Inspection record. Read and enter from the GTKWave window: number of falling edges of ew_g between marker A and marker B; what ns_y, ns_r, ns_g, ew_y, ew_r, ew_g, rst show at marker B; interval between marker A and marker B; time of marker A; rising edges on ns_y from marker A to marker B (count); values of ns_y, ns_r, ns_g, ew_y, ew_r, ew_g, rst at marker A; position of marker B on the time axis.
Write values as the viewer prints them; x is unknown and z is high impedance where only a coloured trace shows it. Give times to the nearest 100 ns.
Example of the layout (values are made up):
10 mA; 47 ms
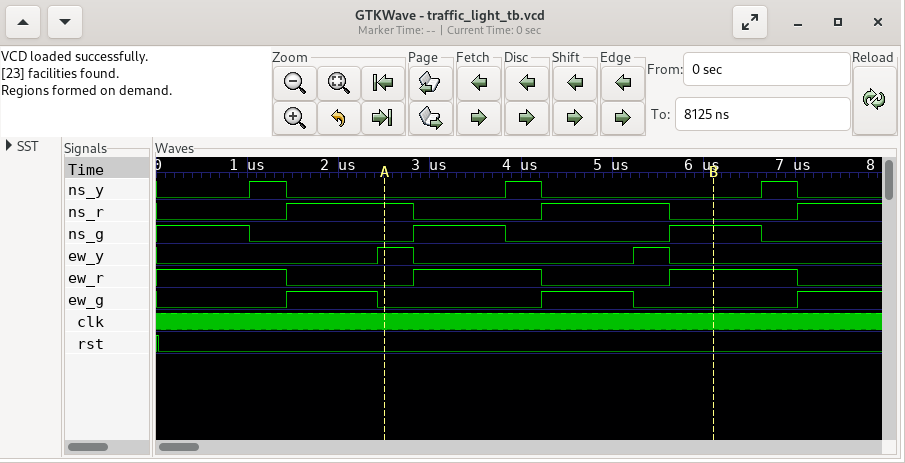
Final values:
1; ns_y=0, ns_r=0, ns_g=1, ew_y=0, ew_r=1, ew_g=0, rst=0; 3600 ns; 2500 ns; 1; ns_y=0, ns_r=1, ns_g=0, ew_y=1, ew_r=0, ew_g=0, rst=0; 6100 ns
